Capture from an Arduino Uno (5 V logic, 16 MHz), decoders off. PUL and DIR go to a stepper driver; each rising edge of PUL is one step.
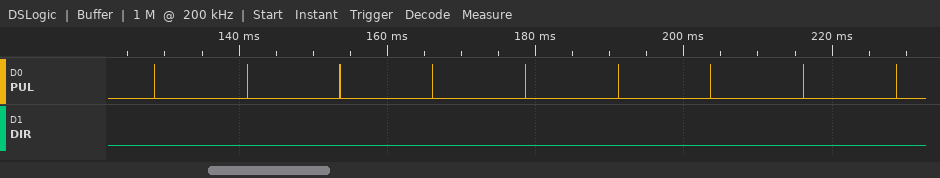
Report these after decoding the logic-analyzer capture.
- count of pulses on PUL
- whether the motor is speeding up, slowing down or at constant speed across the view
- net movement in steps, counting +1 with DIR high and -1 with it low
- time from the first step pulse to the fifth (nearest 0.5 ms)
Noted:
9
constant speed
-9
50.0 ms
